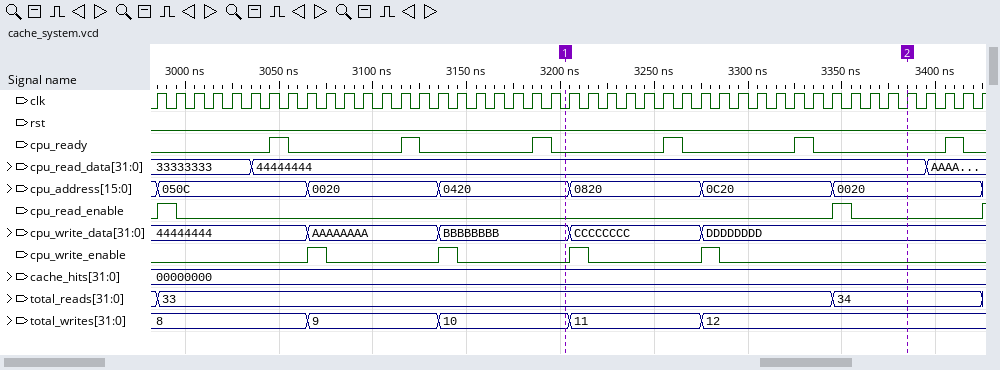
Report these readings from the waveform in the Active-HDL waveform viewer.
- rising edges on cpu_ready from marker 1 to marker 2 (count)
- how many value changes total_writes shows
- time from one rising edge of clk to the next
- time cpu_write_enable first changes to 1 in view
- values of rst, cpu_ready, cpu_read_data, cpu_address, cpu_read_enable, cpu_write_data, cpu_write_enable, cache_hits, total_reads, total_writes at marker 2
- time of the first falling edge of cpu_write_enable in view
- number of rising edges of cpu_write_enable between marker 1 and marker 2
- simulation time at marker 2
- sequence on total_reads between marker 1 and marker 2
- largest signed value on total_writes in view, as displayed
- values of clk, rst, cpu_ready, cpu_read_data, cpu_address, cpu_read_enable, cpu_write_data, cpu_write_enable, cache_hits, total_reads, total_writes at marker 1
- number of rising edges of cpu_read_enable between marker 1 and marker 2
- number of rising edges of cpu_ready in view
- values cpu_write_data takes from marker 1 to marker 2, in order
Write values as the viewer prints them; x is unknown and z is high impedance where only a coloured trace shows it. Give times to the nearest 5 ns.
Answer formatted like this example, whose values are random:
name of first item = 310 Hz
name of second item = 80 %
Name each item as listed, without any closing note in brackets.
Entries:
rising edges on cpu_ready from marker 1 to marker 2 = 2
how many value changes total_writes shows = 4
time from one rising edge of clk to the next = 10 ns
time cpu_write_enable first changes to 1 in view = 3065 ns
values of rst, cpu_ready, cpu_read_data, cpu_address, cpu_read_enable, cpu_write_data, cpu_write_enable, cache_hits, total_reads, total_writes at marker 2 = rst=0, cpu_ready=0, cpu_read_data=44444444, cpu_address=0020, cpu_read_enable=0, cpu_write_data=DDDDDDDD, cpu_write_enable=0, cache_hits=00000000, total_reads=34, total_writes=12
time of the first falling edge of cpu_write_enable in view = 3075 ns
number of rising edges of cpu_write_enable between marker 1 and marker 2 = 2
simulation time at marker 2 = 3385 ns
sequence on total_reads between marker 1 and marker 2 = 33, 34
largest signed value on total_writes in view, as displayed = 12
values of clk, rst, cpu_ready, cpu_read_data, cpu_address, cpu_read_enable, cpu_write_data, cpu_write_enable, cache_hits, total_reads, total_writes at marker 1 = clk=0, rst=0, cpu_ready=0, cpu_read_data=44444444, cpu_address=0420, cpu_read_enable=0, cpu_write_data=BBBBBBBB, cpu_write_enable=0, cache_hits=00000000, total_reads=33, total_writes=10
number of rising edges of cpu_read_enable between marker 1 and marker 2 = 1
number of rising edges of cpu_ready in view = 6
values cpu_write_data takes from marker 1 to marker 2, in order = BBBBBBBB, CCCCCCCC, DDDDDDDD
